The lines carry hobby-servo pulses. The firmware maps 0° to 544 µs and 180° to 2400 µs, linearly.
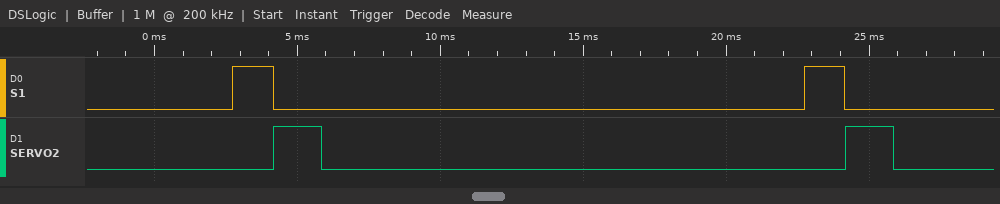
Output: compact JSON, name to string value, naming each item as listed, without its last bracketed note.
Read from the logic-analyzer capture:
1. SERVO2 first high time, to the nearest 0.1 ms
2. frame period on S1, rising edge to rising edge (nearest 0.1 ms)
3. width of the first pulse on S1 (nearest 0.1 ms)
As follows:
{"SERVO2 first high time, to the nearest 0.1 ms": "1.7 ms", "frame period on S1, rising edge to rising edge": "20.0 ms", "width of the first pulse on S1": "1.4 ms"}
